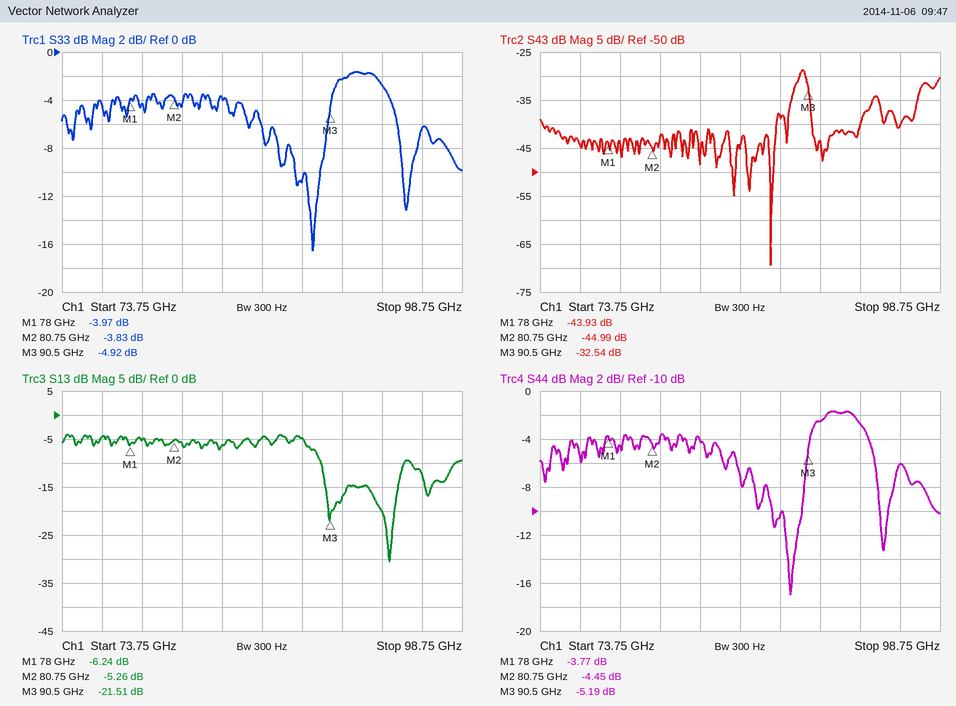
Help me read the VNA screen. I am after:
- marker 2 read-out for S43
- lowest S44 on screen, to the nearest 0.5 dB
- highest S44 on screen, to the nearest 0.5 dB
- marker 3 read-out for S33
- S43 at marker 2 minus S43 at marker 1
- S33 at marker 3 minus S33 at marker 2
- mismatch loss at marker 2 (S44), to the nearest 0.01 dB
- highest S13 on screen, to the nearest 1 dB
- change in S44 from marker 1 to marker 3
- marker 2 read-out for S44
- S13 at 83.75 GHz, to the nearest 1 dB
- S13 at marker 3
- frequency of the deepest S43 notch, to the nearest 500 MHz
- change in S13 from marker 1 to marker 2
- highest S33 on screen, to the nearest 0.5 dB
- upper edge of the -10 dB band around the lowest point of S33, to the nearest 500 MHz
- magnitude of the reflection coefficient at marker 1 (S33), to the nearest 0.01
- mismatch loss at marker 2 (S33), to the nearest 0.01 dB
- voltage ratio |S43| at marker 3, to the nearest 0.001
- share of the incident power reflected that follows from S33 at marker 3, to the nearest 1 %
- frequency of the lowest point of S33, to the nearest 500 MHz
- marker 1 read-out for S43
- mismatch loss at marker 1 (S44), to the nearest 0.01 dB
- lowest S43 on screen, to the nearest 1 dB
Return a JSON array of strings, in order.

["-44.99 dB", "-17.0 dB", "-1.5 dB", "-4.92 dB", "-1.06 dB", "-1.09 dB", "1.93 dB", "-4 dB", "-1.42 dB", "-4.45 dB", "-6 dB", "-21.51 dB", "88.0 GHz", "0.98 dB", "-1.5 dB", "90.0 GHz", "0.63", "2.32 dB", "0.024", "32 %", "89.5 GHz", "-43.93 dB", "2.36 dB", "-69 dB"]
